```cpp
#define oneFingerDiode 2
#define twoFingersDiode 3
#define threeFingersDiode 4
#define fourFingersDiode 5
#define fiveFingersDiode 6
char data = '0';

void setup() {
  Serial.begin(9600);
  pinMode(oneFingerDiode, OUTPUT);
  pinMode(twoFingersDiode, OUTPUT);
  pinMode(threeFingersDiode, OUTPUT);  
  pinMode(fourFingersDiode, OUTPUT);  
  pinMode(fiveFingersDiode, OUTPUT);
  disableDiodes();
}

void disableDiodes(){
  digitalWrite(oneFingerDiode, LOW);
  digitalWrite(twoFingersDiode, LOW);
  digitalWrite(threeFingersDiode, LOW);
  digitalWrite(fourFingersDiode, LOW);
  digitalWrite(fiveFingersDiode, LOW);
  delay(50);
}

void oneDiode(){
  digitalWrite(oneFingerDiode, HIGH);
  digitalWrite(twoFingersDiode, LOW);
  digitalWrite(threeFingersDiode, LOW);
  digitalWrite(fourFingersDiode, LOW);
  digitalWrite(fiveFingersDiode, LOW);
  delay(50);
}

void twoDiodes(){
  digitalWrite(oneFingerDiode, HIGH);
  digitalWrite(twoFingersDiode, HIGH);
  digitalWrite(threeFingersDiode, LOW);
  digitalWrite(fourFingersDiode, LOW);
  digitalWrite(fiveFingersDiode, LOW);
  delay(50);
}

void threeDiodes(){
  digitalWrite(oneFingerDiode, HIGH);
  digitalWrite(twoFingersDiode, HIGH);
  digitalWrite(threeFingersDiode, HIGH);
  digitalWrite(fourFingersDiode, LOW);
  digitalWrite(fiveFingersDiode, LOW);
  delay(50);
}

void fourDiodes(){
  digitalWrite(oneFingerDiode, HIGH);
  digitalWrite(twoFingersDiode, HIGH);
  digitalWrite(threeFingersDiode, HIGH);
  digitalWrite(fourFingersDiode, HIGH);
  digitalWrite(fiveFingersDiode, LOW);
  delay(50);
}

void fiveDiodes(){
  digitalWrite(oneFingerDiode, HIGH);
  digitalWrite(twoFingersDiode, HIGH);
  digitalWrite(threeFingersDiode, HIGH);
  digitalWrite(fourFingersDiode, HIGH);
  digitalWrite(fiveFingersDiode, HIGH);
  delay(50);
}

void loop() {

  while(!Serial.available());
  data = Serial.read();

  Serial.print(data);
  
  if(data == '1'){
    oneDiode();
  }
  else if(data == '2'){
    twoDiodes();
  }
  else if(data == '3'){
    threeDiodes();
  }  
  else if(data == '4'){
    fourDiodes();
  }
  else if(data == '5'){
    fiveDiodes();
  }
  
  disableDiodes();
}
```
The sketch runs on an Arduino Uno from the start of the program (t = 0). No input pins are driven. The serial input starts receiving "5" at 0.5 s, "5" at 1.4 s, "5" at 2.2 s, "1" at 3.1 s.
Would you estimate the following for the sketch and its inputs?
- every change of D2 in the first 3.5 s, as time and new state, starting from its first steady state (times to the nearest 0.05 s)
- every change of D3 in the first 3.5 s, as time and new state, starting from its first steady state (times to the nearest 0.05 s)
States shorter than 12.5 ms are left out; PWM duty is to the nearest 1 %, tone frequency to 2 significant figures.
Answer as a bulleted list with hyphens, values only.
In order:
- 0 s low; 0.5 s high; 0.55 s low; 1.4 s high; 1.45 s low; 2.2 s high; 2.25 s low; 3.1 s high; 3.15 s low
- 0 s low; 0.5 s high; 0.55 s low; 1.4 s high; 1.45 s low; 2.2 s high; 2.25 s low
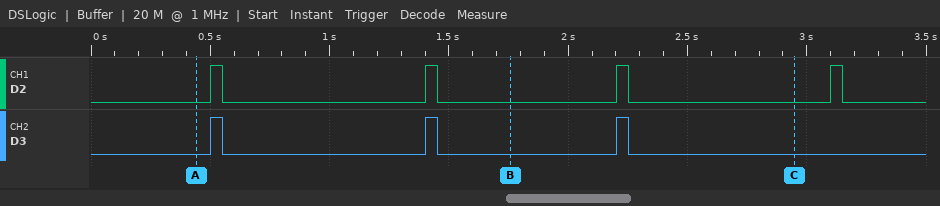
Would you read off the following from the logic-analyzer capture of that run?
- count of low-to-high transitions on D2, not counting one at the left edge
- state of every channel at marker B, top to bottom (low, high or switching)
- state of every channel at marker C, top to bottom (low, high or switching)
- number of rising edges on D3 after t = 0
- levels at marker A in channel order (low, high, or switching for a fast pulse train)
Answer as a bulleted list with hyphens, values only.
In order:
- 4
- D2 low, D3 low
- D2 low, D3 low
- 3
- D2 low, D3 low
